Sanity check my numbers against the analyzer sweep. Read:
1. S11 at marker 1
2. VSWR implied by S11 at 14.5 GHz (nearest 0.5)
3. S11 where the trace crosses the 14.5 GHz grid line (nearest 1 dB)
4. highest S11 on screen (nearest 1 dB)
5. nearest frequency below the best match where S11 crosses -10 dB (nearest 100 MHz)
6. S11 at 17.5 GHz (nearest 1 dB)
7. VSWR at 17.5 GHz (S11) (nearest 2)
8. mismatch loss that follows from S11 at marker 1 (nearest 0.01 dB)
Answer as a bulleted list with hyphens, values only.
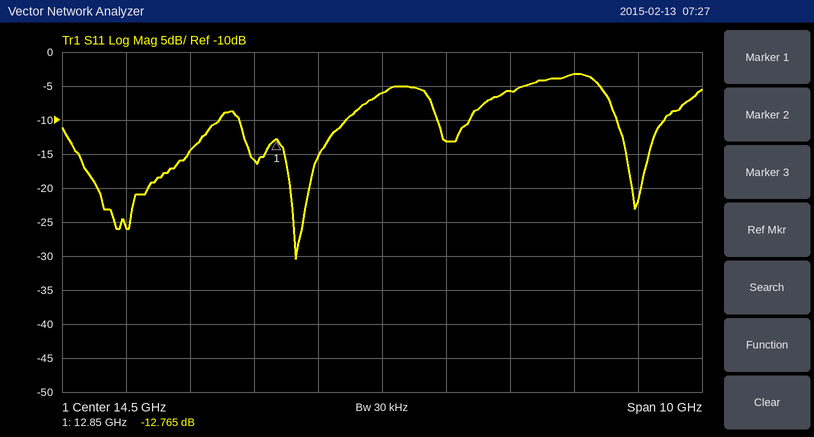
- -12.765 dB
- 3.0
- -6 dB
- -3 dB
- 12.3 GHz
- -3 dB
- 6
- 0.24 dB
